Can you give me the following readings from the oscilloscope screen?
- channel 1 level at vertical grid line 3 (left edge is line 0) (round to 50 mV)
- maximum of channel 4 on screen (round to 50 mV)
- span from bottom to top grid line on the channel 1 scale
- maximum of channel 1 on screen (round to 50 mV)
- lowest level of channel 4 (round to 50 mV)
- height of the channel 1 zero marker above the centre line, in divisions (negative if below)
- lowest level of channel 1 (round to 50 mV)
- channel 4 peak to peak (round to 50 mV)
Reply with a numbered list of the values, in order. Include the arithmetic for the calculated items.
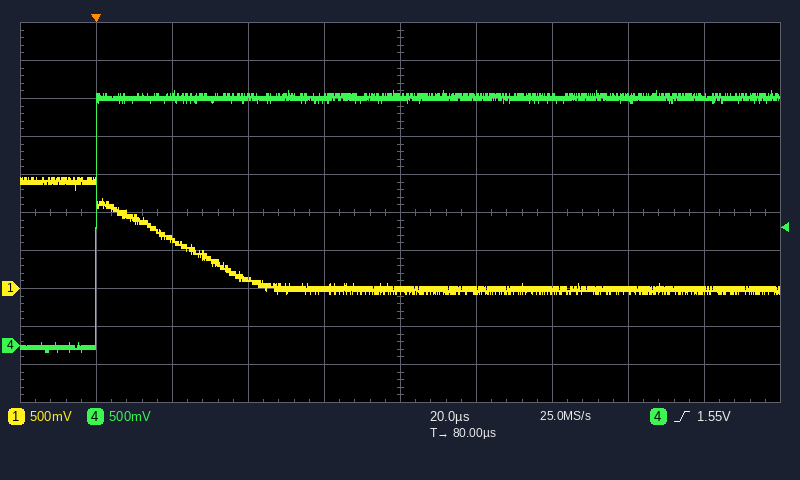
1. 100 mV
2. 3.35 V
3. 5 V
4. 1.45 V
5. -100 mV
6. -2.0 div
7. -50 mV
8. 3.35 V − (-100 mV) = 3.45 V
